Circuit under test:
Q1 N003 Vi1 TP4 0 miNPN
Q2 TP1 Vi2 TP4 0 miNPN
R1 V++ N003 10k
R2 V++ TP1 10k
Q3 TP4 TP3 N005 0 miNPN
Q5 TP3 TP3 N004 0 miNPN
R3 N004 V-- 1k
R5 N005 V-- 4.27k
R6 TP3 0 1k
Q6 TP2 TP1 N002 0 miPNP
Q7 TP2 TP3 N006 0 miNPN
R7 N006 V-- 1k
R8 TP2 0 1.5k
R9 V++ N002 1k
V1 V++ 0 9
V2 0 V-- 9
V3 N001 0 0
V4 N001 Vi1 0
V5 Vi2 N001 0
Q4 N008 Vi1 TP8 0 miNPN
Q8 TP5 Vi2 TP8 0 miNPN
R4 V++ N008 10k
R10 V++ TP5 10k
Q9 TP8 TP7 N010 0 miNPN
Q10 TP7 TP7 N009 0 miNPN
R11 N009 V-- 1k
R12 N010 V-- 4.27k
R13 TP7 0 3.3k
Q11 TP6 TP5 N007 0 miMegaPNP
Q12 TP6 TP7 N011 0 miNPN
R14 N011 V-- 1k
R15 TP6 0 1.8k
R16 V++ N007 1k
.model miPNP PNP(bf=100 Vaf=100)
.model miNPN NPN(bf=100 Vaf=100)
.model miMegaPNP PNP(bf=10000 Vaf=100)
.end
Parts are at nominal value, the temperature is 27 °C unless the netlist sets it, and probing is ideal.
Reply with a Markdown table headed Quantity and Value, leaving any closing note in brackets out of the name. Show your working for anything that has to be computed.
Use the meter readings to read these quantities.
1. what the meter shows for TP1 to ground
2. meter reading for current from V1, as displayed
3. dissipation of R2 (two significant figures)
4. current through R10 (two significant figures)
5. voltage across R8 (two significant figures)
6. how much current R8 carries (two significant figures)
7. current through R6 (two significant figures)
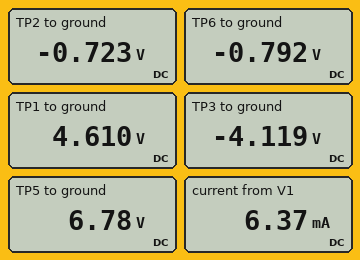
| Quantity | Value |
|---|---|
| what the meter shows for TP1 to ground | 4.610 V |
| meter reading for current from V1, as displayed | 6.37 mA |
| dissipation of R2 | (9 V - 4.61 V)^2 / 10 kΩ = 1.9 mW |
| current through R10 | (9 V - 6.78 V) / 10 kΩ = 220 µA |
| voltage across R8 | 0 V - (-723 mV) = 720 mV |
| how much current R8 carries | (0 V - (-723 mV)) / 1.5 kΩ = 480 µA |
| current through R6 | (0 V - (-4.119 V)) / 1 kΩ = 4.1 mA |
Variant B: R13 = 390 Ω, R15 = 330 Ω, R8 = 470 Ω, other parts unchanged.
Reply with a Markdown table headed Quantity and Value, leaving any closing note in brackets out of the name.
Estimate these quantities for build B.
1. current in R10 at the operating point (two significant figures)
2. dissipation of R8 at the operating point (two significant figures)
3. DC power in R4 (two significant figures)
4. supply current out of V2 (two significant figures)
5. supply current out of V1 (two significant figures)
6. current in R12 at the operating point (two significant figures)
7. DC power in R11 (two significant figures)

| Quantity | Value |
|---|---|
| current in R10 at the operating point | 680 µA |
| dissipation of R8 at the operating point | 110 µW |
| DC power in R4 | 4.6 mW |
| supply current out of V2 | 22 mA |
| supply current out of V1 | 12 mA |
| current in R12 at the operating point | 1.4 mA |
| DC power in R11 | 34 mW |
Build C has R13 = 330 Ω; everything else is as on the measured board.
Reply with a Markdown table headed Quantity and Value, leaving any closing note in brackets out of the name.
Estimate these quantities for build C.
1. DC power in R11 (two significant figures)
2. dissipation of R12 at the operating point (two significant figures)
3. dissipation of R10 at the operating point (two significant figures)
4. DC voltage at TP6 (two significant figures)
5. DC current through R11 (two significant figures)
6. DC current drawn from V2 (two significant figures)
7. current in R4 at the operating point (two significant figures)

| Quantity | Value |
|---|---|
| DC power in R11 | 38 mW |
| dissipation of R12 at the operating point | 8.9 mW |
| dissipation of R10 at the operating point | 5.0 mW |
| DC voltage at TP6 | 330 mV |
| DC current through R11 | 6.1 mA |
| DC current drawn from V2 | 23 mA |
| current in R4 at the operating point | 710 µA |
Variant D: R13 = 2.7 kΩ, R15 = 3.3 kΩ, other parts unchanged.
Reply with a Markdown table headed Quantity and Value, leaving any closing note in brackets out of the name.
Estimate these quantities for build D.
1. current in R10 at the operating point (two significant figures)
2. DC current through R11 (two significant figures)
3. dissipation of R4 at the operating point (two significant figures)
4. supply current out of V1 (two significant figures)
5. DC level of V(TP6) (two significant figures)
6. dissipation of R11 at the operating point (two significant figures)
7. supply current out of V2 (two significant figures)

| Quantity | Value |
|---|---|
| current in R10 at the operating point | 260 µA |
| DC current through R11 | 2.2 mA |
| dissipation of R4 at the operating point | 660 µW |
| supply current out of V1 | 6.8 mA |
| DC level of V(TP6) | -1.3 V |
| dissipation of R11 at the operating point | 4.8 mW |
| supply current out of V2 | 14 mA |
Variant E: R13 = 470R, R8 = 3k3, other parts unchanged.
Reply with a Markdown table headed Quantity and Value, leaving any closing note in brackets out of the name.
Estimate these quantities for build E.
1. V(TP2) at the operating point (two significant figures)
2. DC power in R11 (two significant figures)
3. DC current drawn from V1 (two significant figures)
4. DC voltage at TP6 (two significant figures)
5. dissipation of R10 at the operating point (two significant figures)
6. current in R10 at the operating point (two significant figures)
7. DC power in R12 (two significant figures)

| Quantity | Value |
|---|---|
| V(TP2) at the operating point | -1.6 V |
| DC power in R11 | 31 mW |
| DC current drawn from V1 | 11 mA |
| DC voltage at TP6 | 170 mV |
| dissipation of R10 at the operating point | 4.1 mW |
| current in R10 at the operating point | 640 µA |
| DC power in R12 | 7.3 mW |
